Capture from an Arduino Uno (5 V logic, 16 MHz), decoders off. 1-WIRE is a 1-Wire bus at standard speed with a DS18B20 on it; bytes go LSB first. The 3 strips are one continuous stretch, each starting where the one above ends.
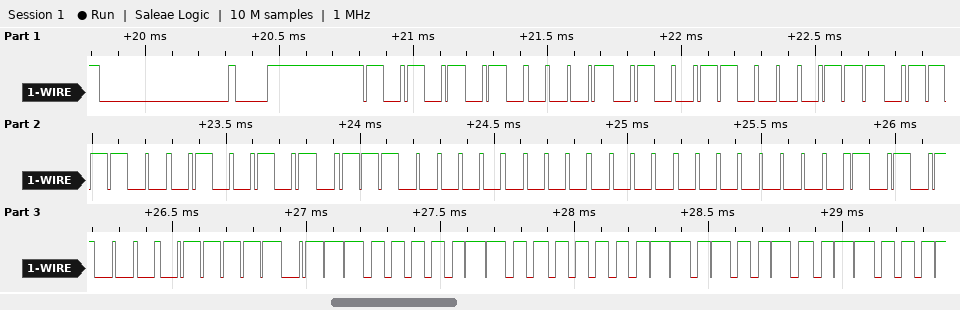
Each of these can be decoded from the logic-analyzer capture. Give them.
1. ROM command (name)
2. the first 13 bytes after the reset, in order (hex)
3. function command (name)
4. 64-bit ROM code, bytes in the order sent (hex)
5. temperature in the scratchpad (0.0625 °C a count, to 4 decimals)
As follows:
Match ROM
55 28 C3 3D 52 07 00 00 15 BE 83 01 4B
Read Scratchpad
28 C3 3D 52 07 00 00 15
24.1875 °C
